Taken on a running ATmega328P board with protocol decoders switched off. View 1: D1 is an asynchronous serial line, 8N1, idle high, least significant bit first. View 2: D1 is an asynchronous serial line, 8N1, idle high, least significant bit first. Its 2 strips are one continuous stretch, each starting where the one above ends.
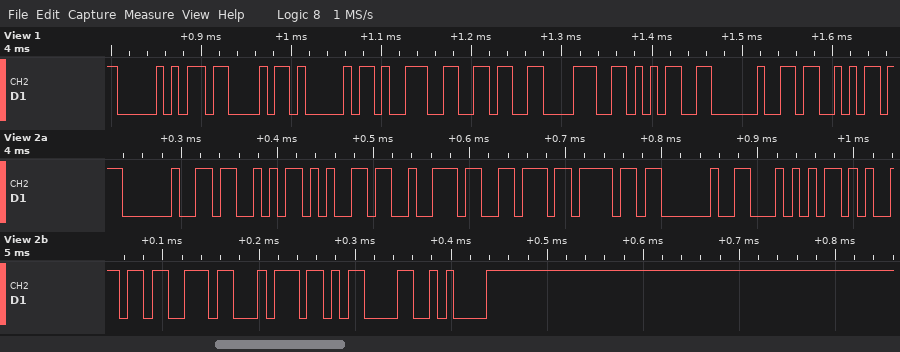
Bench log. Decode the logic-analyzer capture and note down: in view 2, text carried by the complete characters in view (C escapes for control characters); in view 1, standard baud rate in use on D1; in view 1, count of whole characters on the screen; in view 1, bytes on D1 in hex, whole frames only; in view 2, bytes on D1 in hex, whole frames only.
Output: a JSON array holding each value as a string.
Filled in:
["\" Servo Test\\r\\n\"", "115200 baud", "9", "50 43 41 39 36 38 35 20 53", "20 53 65 72 76 6F 20 54 65 73 74 0D 0A"]
